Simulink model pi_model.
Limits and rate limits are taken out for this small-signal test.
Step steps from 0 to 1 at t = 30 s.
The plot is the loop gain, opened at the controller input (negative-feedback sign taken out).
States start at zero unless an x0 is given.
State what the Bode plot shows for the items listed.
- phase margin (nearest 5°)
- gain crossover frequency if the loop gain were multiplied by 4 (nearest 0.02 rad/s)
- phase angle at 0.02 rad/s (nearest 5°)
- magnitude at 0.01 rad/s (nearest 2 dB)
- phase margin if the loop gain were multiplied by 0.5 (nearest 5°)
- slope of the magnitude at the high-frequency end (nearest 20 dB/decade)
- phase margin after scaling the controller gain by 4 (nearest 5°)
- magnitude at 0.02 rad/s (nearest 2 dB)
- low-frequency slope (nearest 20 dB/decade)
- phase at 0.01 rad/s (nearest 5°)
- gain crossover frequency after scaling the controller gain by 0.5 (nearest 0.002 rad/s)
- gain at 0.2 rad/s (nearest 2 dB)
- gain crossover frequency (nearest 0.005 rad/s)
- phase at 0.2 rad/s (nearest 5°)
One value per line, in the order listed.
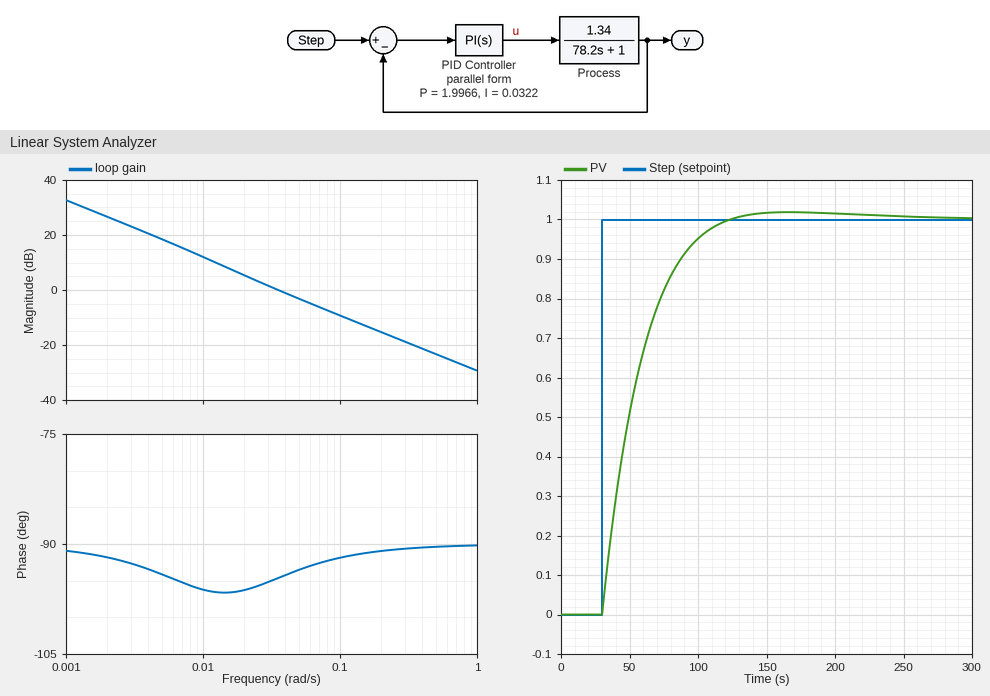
85°
0.14 rad/s
-95°
12 dB
85°
-20 dB/decade
90°
6 dB
-20 dB/decade
-95°
0.018 rad/s
-16 dB
0.035 rad/s
-90°
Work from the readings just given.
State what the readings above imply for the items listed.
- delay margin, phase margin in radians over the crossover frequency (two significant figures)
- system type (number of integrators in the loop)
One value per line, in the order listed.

42 s
1
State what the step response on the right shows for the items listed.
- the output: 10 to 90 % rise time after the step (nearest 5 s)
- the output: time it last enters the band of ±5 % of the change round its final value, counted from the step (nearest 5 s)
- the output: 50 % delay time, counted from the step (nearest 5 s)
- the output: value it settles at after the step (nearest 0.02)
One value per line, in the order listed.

55 s
70 s
20 s
1.00
